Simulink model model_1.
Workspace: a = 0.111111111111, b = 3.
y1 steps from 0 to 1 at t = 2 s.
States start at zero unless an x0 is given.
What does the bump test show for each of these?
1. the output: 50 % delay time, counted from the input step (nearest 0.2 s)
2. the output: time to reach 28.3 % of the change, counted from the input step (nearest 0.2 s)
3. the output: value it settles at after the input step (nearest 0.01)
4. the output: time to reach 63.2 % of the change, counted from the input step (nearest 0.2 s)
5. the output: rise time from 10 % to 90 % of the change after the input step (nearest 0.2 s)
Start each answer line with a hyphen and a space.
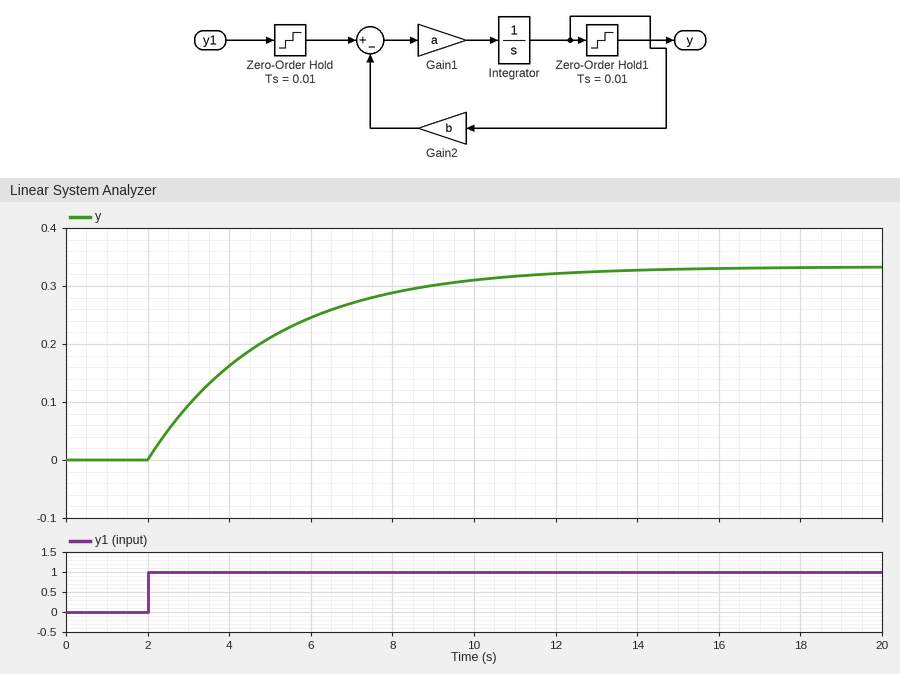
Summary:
- 2.0 s
- 1.0 s
- 0.33
- 3.0 s
- 6.6 s
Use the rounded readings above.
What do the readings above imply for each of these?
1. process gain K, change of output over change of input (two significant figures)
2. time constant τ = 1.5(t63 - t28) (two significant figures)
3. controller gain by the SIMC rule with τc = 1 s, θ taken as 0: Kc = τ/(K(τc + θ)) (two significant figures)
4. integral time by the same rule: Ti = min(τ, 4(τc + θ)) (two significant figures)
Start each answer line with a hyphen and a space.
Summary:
- 0.33
- 3.0 s
- 9.1
- 3.0 s
